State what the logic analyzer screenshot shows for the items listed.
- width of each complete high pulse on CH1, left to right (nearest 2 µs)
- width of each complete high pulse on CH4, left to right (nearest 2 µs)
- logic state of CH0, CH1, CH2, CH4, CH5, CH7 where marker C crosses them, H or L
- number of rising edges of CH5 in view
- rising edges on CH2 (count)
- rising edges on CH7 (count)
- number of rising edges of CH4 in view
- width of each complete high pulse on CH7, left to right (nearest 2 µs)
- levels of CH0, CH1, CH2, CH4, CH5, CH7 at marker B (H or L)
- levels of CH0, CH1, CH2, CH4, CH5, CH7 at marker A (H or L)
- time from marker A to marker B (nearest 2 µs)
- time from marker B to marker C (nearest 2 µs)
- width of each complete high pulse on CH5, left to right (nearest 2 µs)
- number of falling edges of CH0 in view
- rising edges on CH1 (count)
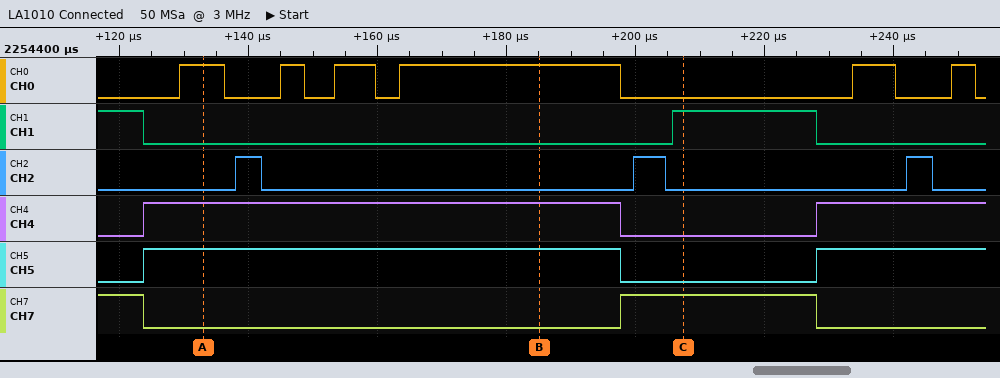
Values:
22 µs
74 µs
CH0=L, CH1=H, CH2=L, CH4=L, CH5=L, CH7=H
2
3
1
2
30 µs
CH0=H, CH1=L, CH2=L, CH4=H, CH5=H, CH7=L
CH0=H, CH1=L, CH2=L, CH4=H, CH5=H, CH7=L
52 µs
22 µs
74 µs
6
1
